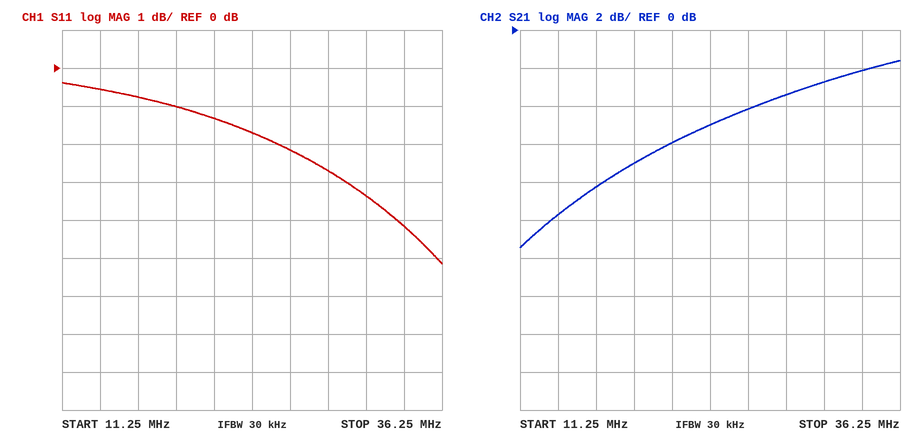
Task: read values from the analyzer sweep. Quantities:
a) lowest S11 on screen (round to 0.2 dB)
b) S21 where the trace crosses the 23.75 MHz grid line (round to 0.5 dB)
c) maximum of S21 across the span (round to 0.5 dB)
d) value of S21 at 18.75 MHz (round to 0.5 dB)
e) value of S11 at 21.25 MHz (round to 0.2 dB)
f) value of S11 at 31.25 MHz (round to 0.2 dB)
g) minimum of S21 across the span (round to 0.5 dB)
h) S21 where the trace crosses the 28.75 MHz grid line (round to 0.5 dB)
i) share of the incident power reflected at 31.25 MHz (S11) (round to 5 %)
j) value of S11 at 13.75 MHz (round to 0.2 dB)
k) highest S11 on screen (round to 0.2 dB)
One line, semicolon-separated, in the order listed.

-5.2 dB; -5.0 dB; -1.5 dB; -7.0 dB; -1.4 dB; -3.4 dB; -11.5 dB; -3.5 dB; 45 %; -0.6 dB; -0.4 dB
